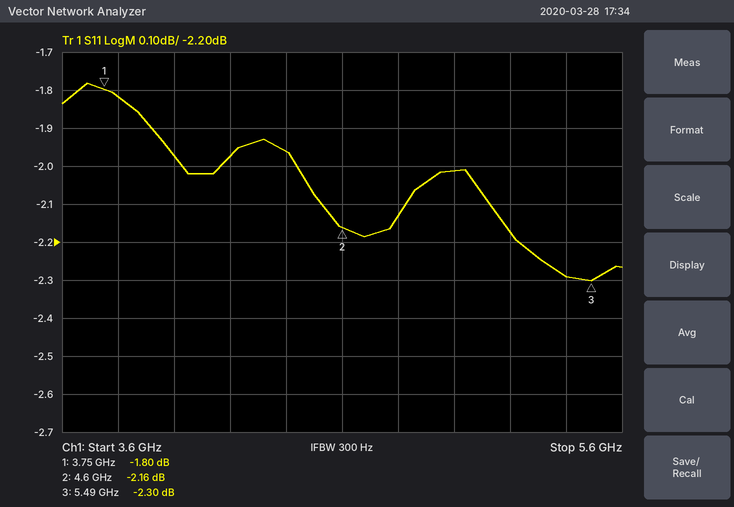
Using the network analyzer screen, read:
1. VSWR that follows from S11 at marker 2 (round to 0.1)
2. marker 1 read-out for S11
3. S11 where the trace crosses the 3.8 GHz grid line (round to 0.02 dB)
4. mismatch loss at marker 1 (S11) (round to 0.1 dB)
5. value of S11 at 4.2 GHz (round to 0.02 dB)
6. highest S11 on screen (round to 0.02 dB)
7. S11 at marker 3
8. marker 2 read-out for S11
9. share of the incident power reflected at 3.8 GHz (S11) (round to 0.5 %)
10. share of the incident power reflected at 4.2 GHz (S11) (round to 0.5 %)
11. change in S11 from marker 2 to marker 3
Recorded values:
8.1
-1.80 dB
-1.82 dB
4.7 dB
-1.98 dB
-1.78 dB
-2.30 dB
-2.16 dB
66.0 %
63.5 %
-0.14 dB
